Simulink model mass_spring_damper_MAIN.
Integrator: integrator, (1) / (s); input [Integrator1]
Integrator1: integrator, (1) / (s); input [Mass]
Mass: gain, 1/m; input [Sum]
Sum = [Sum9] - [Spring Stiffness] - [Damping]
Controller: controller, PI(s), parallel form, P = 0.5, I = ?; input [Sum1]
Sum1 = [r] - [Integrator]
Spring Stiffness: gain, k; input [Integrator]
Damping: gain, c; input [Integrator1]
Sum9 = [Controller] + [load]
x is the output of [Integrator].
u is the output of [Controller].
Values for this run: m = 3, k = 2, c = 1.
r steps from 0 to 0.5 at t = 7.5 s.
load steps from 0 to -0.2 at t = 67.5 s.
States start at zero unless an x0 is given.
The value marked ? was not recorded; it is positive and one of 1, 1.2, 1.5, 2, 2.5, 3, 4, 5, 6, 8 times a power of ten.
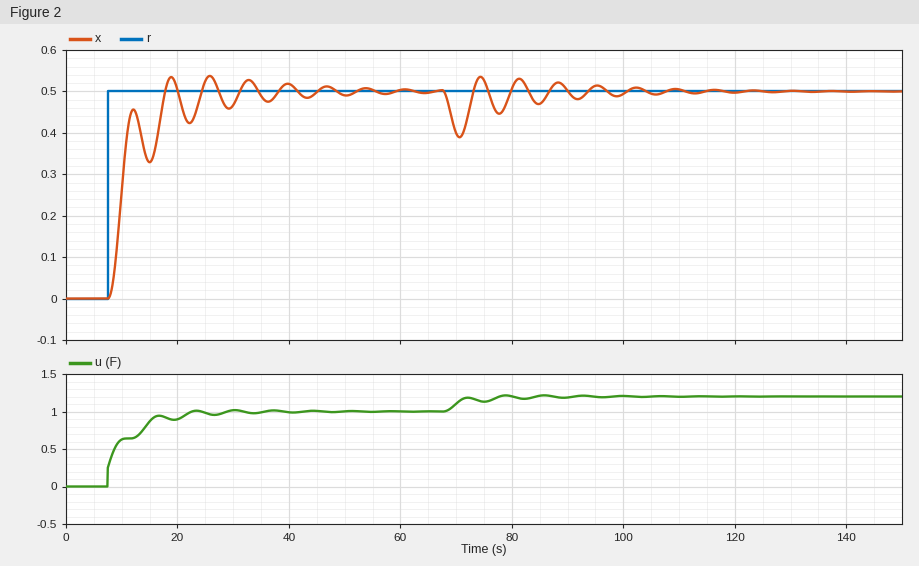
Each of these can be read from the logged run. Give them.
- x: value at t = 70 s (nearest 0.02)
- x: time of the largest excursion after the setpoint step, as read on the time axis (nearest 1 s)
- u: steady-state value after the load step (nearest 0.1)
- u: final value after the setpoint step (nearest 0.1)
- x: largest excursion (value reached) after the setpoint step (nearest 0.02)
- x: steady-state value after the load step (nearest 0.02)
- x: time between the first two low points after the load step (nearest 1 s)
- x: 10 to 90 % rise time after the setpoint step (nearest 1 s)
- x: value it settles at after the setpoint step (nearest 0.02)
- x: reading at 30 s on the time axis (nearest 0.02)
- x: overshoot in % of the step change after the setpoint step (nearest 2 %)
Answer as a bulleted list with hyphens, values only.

- 0.40
- 26 s
- 1.2
- 1.0
- 0.54
- 0.50
- 7 s
- 3 s
- 0.50
- 0.46
- 8 %
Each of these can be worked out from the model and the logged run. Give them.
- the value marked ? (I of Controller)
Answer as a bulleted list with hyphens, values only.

- 0.5
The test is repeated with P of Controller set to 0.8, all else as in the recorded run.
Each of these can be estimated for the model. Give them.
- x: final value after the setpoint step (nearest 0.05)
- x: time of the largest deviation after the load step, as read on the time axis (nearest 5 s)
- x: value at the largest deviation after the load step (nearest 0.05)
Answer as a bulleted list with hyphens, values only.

- 0.50
- 70 s
- 0.40
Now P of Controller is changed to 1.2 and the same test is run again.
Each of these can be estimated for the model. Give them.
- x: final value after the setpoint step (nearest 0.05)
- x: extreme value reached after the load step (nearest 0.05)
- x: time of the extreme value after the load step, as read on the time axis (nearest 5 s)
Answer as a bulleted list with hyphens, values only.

- 0.50
- 0.40
- 70 s
